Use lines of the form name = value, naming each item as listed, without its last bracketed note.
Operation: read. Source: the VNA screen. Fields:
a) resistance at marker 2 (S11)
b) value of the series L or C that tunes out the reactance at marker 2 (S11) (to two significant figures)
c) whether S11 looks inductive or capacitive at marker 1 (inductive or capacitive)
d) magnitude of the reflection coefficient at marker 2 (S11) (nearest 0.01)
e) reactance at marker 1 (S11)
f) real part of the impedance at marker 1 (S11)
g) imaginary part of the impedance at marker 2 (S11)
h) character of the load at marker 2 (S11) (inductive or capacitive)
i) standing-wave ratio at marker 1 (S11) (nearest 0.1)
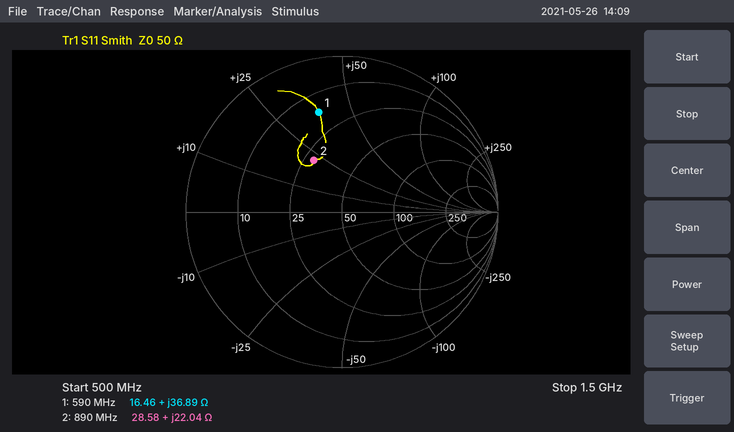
resistance at marker 2 = 28.58 Ω
value of the series L or C that tunes out the reactance at marker 2 (S11) = 8.1 pF
whether S11 looks inductive or capacitive at marker 1 = inductive
magnitude of the reflection coefficient at marker 2 (S11) = 0.38
reactance at marker 1 = +36.89 Ω
real part of the impedance at marker 1 = 16.46 Ω
imaginary part of the impedance at marker 2 = +22.04 Ω
character of the load at marker 2 (S11) = inductive
standing-wave ratio at marker 1 (S11) = 4.8
